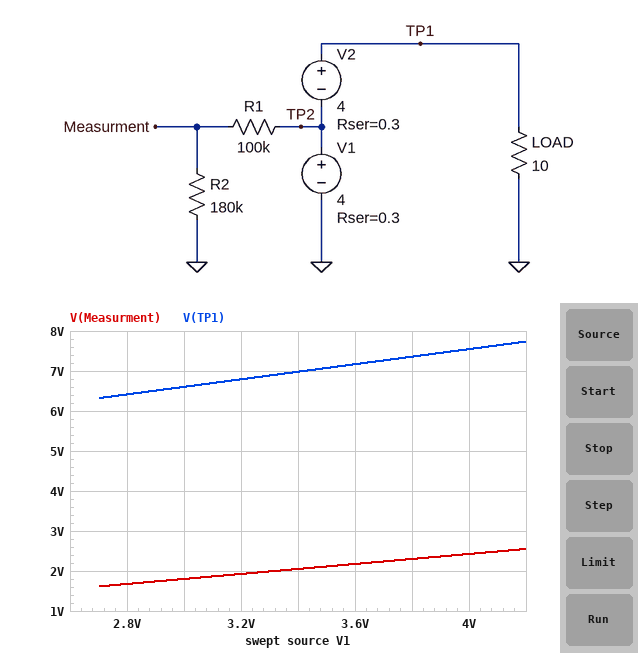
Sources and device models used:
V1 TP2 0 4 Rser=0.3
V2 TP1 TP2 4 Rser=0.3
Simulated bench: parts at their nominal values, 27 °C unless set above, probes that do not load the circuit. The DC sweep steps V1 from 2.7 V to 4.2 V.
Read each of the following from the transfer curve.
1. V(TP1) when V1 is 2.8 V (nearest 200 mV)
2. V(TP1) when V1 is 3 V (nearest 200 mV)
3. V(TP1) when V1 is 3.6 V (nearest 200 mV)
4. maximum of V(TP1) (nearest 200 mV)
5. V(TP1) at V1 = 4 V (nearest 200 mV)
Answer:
6.4 V
6.6 V
7.2 V
7.8 V
7.6 V
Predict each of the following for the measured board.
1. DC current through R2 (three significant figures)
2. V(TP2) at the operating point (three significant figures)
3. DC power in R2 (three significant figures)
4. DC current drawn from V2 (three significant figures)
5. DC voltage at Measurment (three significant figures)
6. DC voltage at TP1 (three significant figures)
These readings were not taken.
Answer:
13.5 µA
3.77 V
32.7 µW
755 mA
2.43 V
7.55 V
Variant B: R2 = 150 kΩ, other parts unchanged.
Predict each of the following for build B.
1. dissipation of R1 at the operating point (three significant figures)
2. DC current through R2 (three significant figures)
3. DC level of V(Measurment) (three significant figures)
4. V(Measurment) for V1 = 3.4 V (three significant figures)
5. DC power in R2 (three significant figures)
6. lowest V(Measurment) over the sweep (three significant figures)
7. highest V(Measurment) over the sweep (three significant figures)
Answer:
22.8 µW
15.1 µA
2.26 V
1.91 V
34.2 µW
1.51 V
2.38 V
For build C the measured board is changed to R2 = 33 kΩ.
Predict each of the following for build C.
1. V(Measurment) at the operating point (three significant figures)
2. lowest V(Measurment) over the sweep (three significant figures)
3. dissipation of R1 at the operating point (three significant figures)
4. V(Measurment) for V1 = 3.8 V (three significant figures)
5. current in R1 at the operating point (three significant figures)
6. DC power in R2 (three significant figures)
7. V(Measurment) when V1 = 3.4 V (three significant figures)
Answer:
936 mV
623 mV
80.5 µW
888 mV
28.4 µA
26.6 µW
792 mV
